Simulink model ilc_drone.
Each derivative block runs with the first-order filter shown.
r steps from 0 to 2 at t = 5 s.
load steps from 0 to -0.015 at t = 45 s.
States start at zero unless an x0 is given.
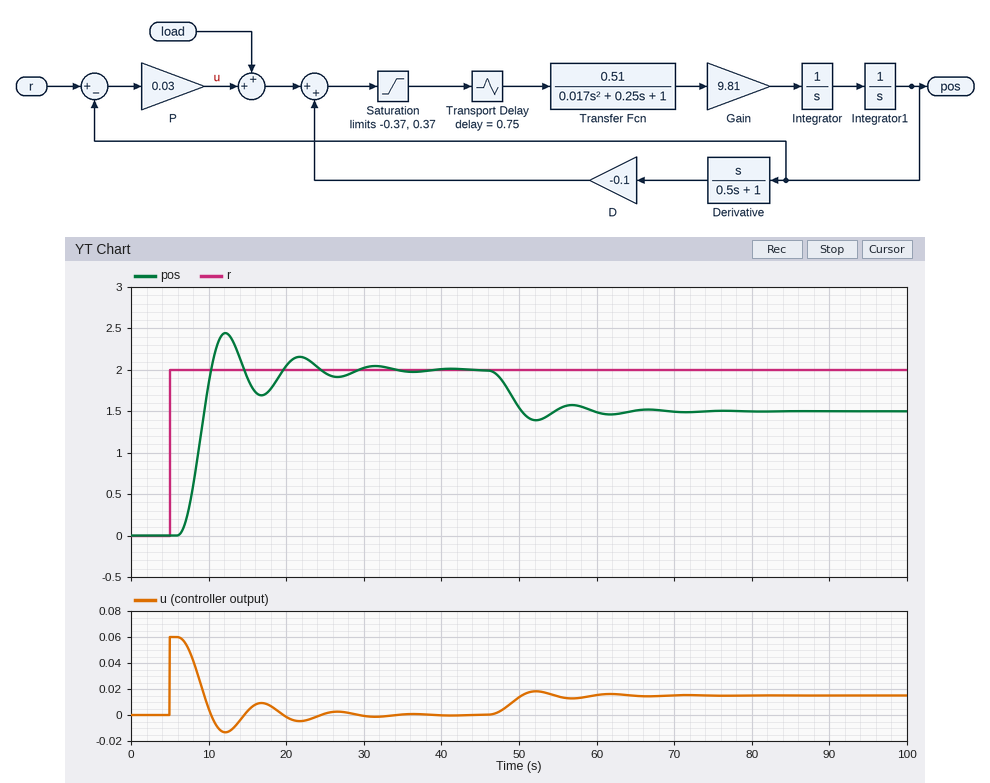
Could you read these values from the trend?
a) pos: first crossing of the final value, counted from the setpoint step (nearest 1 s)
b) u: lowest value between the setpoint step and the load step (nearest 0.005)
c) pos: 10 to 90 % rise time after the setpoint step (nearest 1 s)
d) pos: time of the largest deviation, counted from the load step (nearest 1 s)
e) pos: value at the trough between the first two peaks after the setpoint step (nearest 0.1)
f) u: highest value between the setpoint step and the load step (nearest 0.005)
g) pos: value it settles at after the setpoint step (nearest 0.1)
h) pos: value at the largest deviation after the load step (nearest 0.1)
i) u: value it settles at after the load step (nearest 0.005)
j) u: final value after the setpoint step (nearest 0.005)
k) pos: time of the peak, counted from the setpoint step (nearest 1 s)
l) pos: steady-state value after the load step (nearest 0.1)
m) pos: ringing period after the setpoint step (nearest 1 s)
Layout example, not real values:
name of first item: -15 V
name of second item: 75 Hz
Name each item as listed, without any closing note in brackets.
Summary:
pos: first crossing of the final value, counted from the setpoint step: 5 s
u: lowest value between the setpoint step and the load step: -0.015
pos: 10 to 90 % rise time after the setpoint step: 3 s
pos: time of the largest deviation, counted from the load step: 7 s
pos: value at the trough between the first two peaks after the setpoint step: 1.7
u: highest value between the setpoint step and the load step: 0.060
pos: value it settles at after the setpoint step: 2.0
pos: value at the largest deviation after the load step: 1.4
u: value it settles at after the load step: 0.015
u: final value after the setpoint step: 0.000
pos: time of the peak, counted from the setpoint step: 7 s
pos: steady-state value after the load step: 1.5
pos: ringing period after the setpoint step: 10 s
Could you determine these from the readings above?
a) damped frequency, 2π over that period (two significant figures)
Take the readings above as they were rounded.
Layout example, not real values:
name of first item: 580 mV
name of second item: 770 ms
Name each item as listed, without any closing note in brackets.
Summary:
damped frequency, 2π over that period: 0.63 rad/s
